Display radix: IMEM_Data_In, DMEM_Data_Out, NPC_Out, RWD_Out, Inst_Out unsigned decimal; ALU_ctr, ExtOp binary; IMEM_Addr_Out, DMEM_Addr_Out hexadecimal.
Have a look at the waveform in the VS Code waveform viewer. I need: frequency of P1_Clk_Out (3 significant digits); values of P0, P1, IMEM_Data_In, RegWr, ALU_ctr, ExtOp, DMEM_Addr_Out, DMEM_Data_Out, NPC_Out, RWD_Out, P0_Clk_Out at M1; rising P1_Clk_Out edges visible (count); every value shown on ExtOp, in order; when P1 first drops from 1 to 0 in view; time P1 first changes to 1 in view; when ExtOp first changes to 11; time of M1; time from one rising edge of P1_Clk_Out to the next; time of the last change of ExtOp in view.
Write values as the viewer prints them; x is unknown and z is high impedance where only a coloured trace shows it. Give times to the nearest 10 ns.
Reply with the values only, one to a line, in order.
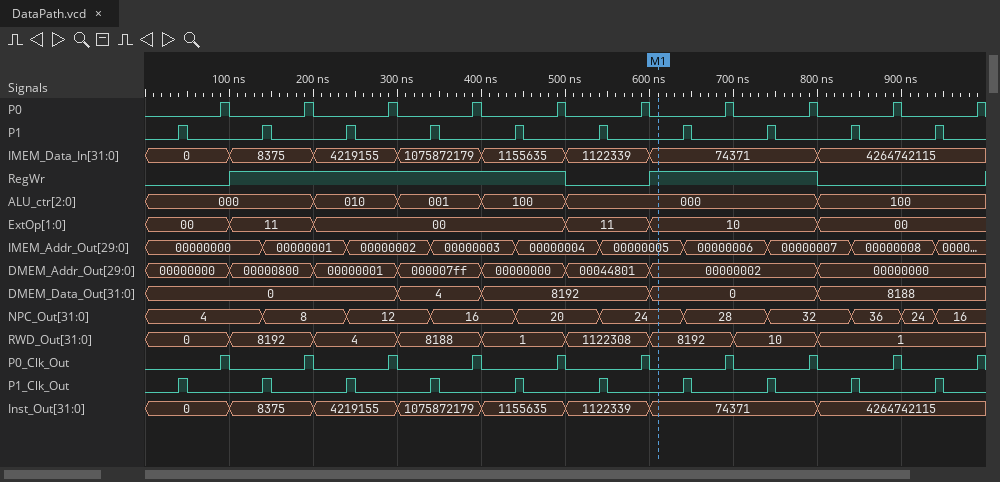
10.0 MHz
P0=0, P1=0, IMEM_Data_In=74371, RegWr=1, ALU_ctr=000, ExtOp=10, DMEM_Addr_Out=00000002, DMEM_Data_Out=0, NPC_Out=24, RWD_Out=8192, P0_Clk_Out=0
10
00, 11, 00, 11, 10, 00
50 ns
40 ns
100 ns
610 ns
100 ns
800 ns
